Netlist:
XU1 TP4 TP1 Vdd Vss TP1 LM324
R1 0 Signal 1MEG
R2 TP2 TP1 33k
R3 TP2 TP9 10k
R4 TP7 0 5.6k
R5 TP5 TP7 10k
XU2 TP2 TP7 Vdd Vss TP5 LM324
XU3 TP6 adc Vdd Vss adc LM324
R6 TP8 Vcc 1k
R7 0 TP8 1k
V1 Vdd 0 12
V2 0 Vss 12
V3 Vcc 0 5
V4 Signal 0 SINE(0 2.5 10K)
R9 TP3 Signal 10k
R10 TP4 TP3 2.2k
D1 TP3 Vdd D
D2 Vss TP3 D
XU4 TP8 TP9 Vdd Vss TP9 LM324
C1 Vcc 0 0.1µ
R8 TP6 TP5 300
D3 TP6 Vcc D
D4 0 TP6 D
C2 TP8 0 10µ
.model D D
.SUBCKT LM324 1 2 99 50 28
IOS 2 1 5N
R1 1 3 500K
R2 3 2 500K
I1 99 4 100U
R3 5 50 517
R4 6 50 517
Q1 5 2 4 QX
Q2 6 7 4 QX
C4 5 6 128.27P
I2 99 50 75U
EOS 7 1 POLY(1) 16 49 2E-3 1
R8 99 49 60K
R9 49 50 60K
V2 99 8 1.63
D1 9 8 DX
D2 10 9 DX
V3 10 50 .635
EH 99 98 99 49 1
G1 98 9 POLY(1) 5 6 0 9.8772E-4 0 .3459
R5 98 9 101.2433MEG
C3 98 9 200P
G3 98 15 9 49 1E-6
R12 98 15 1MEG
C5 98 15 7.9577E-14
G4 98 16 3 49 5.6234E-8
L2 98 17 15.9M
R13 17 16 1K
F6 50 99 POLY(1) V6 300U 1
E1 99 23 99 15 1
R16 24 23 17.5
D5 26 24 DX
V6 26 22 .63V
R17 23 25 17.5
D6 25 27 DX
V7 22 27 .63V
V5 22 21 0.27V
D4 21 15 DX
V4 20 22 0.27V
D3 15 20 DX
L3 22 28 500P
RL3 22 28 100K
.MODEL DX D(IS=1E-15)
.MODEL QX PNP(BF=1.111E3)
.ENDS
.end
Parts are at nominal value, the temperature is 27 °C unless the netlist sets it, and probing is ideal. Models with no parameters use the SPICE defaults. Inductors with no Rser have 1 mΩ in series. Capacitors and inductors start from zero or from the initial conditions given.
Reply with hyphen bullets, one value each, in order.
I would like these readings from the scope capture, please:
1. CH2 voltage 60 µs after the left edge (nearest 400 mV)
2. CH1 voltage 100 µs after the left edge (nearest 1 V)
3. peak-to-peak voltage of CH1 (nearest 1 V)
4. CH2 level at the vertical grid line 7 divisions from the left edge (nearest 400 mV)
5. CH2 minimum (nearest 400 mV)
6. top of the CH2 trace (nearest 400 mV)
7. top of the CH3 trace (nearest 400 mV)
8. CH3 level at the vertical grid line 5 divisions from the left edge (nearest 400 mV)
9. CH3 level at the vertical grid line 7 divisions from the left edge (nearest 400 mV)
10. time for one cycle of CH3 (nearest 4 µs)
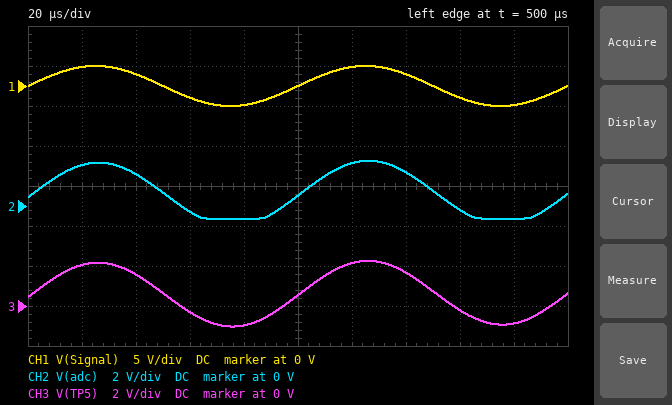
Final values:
- -400 mV
- 0 V
- 5 V
- 1.6 V
- -800 mV
- 2.4 V
- 2.4 V
- 400 mV
- 1.6 V
- 100 µs
